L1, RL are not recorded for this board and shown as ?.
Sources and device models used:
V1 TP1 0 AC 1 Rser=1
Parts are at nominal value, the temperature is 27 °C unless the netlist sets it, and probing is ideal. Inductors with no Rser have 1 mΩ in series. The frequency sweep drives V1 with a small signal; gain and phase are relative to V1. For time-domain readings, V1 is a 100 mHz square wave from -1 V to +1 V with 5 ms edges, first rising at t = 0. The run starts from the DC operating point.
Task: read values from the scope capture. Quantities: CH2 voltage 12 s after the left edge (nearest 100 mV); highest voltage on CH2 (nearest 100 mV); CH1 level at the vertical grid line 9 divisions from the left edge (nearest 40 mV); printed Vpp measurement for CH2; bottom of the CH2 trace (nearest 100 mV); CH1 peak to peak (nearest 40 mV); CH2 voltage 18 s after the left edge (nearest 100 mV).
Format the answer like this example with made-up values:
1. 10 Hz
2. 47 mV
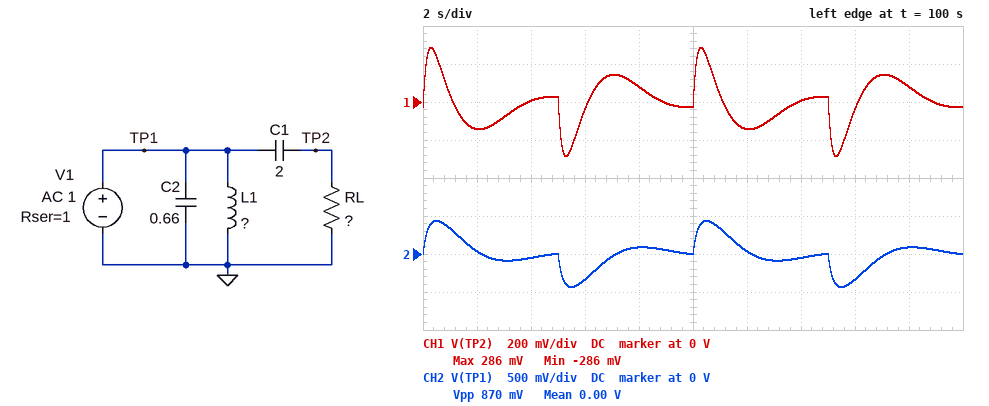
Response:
1. 0 V
2. 400 mV
3. 80 mV
4. 870 mV
5. -400 mV
6. 560 mV
7. 100 mV
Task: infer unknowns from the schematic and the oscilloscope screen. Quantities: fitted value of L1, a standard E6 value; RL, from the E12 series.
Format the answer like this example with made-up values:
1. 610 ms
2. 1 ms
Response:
1. 220 mH
2. 0.33 Ω
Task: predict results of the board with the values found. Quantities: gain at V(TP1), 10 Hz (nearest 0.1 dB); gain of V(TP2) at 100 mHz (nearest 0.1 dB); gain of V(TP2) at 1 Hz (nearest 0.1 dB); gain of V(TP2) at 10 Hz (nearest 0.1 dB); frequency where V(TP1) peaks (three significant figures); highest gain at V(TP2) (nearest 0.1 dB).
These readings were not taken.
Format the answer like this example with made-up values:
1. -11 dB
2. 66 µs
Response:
1. -32.4 dB
2. -23.8 dB
3. -15.3 dB
4. -32.4 dB
5. 222 mHz
6. -11.1 dB
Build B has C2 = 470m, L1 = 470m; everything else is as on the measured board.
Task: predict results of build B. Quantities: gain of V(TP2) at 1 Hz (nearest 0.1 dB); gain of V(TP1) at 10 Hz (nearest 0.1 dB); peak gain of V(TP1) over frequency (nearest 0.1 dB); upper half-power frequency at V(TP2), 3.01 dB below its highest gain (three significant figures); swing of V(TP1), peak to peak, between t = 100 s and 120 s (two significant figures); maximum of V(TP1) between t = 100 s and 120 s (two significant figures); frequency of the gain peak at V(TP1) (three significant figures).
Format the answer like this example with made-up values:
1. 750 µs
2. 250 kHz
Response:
1. -14.4 dB
2. -29.5 dB
3. -5.6 dB
4. 823 mHz
5. 1.3 V
6. 670 mV
7. 143 mHz
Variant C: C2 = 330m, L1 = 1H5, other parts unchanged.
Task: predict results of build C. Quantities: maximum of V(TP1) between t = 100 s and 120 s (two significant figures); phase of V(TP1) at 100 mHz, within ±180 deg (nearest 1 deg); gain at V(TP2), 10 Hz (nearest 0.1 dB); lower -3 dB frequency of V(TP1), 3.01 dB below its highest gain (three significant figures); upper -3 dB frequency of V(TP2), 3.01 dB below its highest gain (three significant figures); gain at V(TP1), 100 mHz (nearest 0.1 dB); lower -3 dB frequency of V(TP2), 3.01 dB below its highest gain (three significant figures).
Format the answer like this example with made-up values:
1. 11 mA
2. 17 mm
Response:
1. 790 mV
2. -9 deg
3. -26.5 dB
4. 48.5 mHz
5. 1.51 Hz
6. -3.3 dB
7. 65.5 mHz
